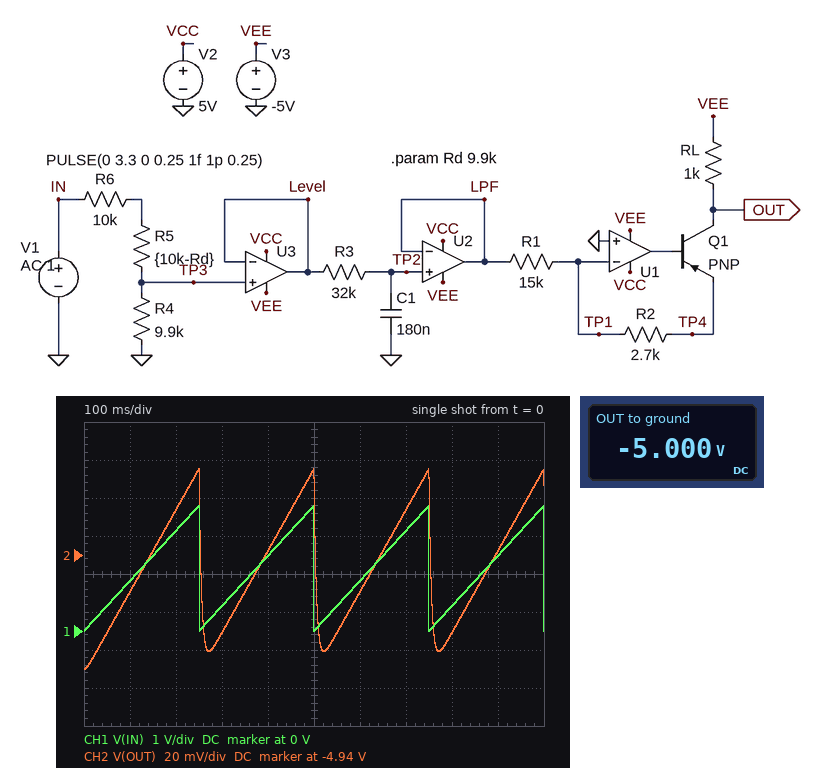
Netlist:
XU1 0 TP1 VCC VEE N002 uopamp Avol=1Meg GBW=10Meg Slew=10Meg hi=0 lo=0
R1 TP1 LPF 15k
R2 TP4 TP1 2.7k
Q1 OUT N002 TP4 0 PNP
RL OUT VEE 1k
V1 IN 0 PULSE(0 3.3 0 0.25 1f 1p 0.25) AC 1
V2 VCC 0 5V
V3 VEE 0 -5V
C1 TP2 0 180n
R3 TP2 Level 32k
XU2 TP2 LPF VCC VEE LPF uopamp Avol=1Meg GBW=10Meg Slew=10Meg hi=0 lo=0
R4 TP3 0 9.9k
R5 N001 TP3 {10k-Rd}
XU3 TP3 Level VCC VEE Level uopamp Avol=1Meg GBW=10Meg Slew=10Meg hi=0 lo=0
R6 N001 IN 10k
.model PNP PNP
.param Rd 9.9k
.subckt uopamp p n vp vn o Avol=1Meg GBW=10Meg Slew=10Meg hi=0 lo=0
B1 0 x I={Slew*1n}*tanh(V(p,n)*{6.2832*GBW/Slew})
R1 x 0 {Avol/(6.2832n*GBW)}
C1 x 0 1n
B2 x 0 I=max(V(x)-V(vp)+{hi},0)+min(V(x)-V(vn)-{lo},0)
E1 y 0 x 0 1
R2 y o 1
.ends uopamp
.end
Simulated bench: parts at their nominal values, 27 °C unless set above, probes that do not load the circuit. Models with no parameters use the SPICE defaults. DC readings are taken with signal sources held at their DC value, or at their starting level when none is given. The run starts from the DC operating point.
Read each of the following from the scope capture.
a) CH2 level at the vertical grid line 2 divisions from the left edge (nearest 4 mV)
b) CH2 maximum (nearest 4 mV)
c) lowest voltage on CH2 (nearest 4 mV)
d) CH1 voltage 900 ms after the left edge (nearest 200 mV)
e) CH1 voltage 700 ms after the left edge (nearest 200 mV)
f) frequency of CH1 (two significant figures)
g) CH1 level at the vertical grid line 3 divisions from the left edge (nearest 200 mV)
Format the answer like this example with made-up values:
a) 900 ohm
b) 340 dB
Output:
a) -4.916 V
b) -4.896 V
c) -5.000 V
d) 2.0 V
e) 2.6 V
f) 4.0 Hz
g) 600 mV
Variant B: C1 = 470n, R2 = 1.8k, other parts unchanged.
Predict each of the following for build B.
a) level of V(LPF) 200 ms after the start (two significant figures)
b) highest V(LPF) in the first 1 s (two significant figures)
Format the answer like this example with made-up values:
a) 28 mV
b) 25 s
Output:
a) 1.2 V
b) 1.5 V
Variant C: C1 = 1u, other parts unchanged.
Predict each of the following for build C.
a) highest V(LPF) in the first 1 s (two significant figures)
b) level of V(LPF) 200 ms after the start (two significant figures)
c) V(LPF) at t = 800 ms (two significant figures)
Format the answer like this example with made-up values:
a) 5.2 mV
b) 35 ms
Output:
a) 1.4 V
b) 1.1 V
c) 460 mV
